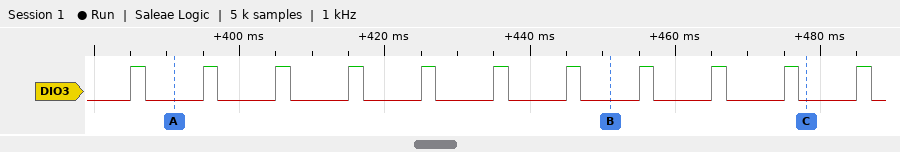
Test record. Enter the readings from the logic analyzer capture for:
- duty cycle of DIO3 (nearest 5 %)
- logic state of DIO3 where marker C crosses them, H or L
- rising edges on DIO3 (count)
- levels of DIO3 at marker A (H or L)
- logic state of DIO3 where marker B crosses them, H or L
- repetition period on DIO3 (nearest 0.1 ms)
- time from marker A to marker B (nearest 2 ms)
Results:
20 %
DIO3=L
11
DIO3=L
DIO3=L
10 ms
60 ms
